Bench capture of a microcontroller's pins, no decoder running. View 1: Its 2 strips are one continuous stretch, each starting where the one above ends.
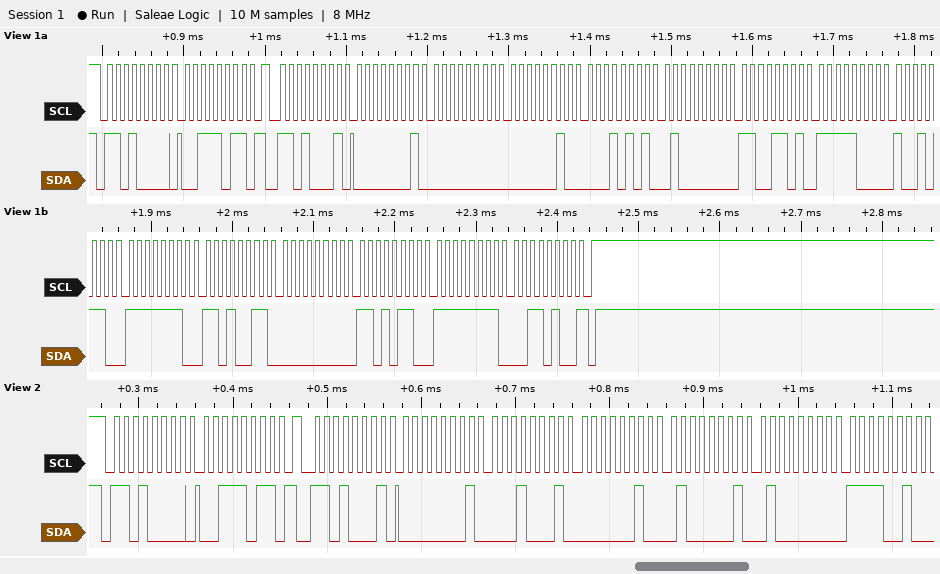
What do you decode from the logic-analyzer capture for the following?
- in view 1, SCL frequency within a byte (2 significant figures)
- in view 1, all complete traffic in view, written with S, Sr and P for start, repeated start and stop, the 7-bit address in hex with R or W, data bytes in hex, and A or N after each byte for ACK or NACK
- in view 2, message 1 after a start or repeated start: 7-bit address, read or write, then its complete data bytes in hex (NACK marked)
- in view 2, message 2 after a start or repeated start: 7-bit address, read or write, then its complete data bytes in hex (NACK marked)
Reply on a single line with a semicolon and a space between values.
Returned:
100 kHz; S 68W A 3B A Sr 68R A 01 A 00 A 02 A 15 A 40 A CD A F8 A 96 A FE A D3 A 00 A D6 A FF A 34 N P; 0x68 write: 3B; 0x68 read: 01 11 02 41 40 F2
